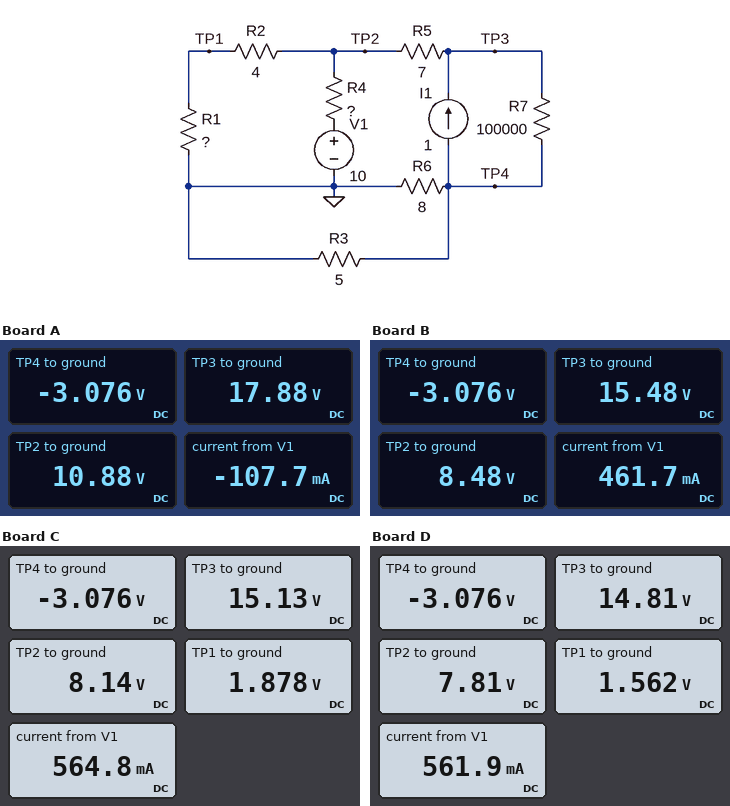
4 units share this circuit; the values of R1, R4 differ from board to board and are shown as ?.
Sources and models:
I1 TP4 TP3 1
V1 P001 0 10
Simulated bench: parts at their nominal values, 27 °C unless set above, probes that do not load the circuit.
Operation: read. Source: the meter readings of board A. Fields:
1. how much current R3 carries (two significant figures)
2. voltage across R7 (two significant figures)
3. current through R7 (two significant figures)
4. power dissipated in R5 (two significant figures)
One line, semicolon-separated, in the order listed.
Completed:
620 mA; 21 V; 210 µA; 7.0 W
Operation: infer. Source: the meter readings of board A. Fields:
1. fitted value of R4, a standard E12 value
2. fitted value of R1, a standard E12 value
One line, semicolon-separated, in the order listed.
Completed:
8.2 Ω; 8.2 Ω
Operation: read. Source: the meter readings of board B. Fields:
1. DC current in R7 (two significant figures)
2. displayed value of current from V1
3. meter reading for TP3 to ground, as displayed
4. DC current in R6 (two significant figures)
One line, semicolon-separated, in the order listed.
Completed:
190 µA; 461.7 mA; 15.48 V; 380 mA
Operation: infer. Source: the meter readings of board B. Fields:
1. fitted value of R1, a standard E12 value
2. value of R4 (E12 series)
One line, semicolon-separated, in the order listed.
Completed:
1.8 Ω; 3.3 Ω
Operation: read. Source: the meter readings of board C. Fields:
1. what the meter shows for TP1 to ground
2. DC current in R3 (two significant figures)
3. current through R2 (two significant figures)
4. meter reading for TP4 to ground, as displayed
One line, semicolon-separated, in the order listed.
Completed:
1.878 V; 620 mA; 1.6 A; -3.076 V
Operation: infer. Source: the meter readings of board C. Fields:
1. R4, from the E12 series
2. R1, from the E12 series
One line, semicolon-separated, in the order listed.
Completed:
3.3 Ω; 1.2 Ω
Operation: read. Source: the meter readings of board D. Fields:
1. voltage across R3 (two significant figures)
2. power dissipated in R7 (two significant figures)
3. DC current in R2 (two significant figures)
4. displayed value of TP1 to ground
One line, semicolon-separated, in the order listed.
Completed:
3.1 V; 3.2 mW; 1.6 A; 1.562 V
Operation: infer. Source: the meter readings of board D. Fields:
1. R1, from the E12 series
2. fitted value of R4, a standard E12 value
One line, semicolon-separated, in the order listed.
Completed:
1 Ω; 3.9 Ω
